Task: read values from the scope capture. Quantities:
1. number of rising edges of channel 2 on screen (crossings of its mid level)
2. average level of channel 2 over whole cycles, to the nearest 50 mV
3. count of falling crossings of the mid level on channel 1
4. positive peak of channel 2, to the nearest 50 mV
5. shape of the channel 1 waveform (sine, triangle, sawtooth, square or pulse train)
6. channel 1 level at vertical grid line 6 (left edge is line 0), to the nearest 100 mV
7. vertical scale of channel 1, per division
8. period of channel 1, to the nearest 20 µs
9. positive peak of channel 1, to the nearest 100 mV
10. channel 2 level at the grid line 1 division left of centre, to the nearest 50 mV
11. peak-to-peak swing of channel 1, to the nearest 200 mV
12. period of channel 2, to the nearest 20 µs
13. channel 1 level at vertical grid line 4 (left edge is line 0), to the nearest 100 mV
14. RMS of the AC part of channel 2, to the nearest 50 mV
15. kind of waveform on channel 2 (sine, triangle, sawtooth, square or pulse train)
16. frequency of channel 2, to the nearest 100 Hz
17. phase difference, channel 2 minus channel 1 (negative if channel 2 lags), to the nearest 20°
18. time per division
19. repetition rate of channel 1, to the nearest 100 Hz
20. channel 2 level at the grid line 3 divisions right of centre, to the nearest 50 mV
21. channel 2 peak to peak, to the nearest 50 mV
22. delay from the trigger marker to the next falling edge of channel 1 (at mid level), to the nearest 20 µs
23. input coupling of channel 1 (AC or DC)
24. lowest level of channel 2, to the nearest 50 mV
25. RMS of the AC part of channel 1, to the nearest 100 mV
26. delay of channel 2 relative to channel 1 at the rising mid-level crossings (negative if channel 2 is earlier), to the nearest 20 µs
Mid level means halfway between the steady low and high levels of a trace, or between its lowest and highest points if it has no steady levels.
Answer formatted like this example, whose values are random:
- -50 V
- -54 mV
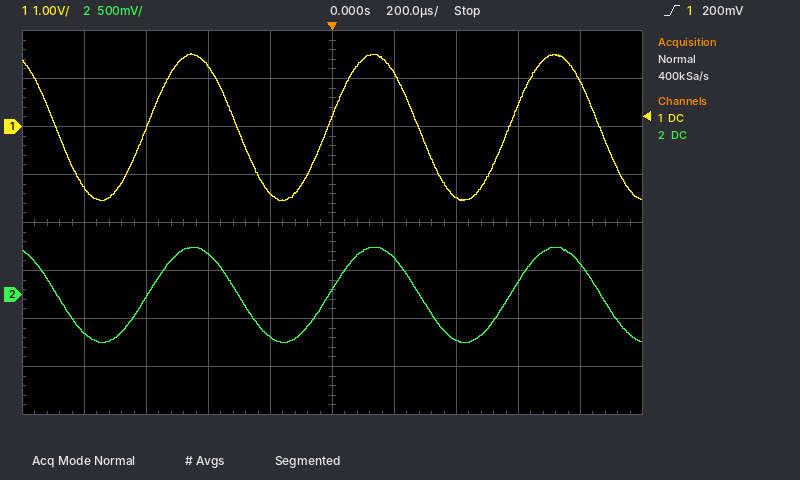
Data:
- 3
- 0 mV
- 4
- 500 mV
- sine
- 1.1 V
- 1 V
- 580 µs
- 1.5 V
- -450 mV
- 3.0 V
- 580 µs
- -1.4 V
- 350 mV
- sine
- 1.7 kHz
- 0°
- 200 µs
- 1.7 kHz
- 150 mV
- 1.00 V
- 280 µs
- DC
- -500 mV
- 1.1 V
- 0 µs
